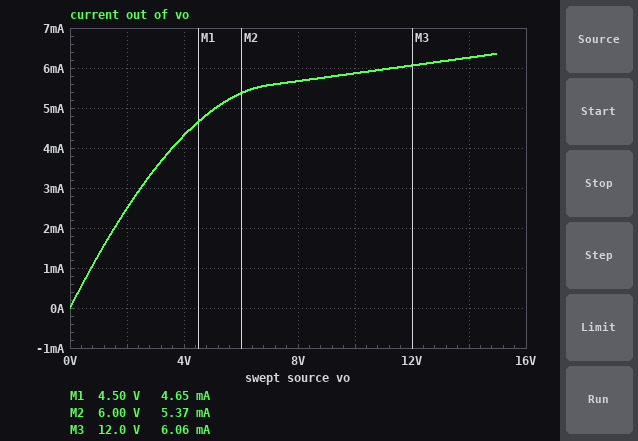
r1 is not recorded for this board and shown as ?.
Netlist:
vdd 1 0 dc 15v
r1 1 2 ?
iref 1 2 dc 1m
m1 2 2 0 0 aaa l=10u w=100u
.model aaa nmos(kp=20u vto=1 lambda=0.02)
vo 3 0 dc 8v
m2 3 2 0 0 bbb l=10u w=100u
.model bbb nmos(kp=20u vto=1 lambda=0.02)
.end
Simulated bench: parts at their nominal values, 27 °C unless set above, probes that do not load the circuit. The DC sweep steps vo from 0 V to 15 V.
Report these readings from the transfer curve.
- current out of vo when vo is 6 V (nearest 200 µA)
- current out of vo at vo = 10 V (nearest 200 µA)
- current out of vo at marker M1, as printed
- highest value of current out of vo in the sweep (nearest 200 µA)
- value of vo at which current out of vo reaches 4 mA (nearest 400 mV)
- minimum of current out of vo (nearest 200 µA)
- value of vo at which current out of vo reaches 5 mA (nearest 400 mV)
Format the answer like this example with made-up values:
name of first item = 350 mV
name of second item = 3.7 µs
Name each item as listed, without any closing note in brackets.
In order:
current out of vo when vo is 6 V = 5.4 mA
current out of vo at vo = 10 V = 5.8 mA
current out of vo at marker M1, as printed = 4.65 mA
highest value of current out of vo in the sweep = 6.4 mA
value of vo at which current out of vo reaches 4 mA = 3.6 V
minimum of current out of vo = 0 A
value of vo at which current out of vo reaches 5 mA = 5.2 V
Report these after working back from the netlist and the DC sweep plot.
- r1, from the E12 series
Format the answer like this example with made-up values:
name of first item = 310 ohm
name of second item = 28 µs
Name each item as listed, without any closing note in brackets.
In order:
r1, from the E12 series = 1.5 kΩ
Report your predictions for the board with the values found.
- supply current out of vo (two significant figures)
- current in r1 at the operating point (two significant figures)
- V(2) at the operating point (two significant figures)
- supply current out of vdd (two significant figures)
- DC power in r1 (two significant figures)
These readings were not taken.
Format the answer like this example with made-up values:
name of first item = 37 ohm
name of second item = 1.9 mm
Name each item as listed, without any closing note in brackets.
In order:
supply current out of vo = 5.7 mA
current in r1 at the operating point = 4.7 mA
V(2) at the operating point = 8.0 V
supply current out of vdd = 5.7 mA
DC power in r1 = 33 mW
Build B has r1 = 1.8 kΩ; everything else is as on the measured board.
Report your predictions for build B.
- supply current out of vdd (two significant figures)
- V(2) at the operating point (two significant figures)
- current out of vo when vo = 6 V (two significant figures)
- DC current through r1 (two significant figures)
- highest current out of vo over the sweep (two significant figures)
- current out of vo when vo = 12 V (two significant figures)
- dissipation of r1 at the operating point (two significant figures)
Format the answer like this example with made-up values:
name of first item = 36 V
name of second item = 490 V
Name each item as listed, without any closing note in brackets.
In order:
supply current out of vdd = 5.1 mA
V(2) at the operating point = 7.6 V
current out of vo when vo = 6 V = 4.9 mA
DC current through r1 = 4.1 mA
highest current out of vo over the sweep = 5.7 mA
current out of vo when vo = 12 V = 5.5 mA
dissipation of r1 at the operating point = 30 mW
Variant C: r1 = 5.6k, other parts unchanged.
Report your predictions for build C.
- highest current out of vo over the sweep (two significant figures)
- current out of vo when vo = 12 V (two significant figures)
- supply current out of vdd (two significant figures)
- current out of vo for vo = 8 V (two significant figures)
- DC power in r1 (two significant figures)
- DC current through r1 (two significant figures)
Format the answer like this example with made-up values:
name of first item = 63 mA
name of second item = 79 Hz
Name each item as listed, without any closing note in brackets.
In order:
highest current out of vo over the sweep = 3.1 mA
current out of vo when vo = 12 V = 2.9 mA
supply current out of vdd = 2.6 mA
current out of vo for vo = 8 V = 2.7 mA
DC power in r1 = 15 mW
DC current through r1 = 1.6 mA
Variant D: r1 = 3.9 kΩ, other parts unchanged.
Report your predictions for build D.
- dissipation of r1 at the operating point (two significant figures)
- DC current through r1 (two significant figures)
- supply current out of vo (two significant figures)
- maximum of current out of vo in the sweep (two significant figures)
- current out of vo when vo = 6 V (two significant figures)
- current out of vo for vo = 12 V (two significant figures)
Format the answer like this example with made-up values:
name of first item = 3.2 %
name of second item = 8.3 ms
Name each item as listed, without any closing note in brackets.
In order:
dissipation of r1 at the operating point = 19 mW
DC current through r1 = 2.2 mA
supply current out of vo = 3.3 mA
maximum of current out of vo in the sweep = 3.7 mA
current out of vo when vo = 6 V = 3.2 mA
current out of vo for vo = 12 V = 3.5 mA
